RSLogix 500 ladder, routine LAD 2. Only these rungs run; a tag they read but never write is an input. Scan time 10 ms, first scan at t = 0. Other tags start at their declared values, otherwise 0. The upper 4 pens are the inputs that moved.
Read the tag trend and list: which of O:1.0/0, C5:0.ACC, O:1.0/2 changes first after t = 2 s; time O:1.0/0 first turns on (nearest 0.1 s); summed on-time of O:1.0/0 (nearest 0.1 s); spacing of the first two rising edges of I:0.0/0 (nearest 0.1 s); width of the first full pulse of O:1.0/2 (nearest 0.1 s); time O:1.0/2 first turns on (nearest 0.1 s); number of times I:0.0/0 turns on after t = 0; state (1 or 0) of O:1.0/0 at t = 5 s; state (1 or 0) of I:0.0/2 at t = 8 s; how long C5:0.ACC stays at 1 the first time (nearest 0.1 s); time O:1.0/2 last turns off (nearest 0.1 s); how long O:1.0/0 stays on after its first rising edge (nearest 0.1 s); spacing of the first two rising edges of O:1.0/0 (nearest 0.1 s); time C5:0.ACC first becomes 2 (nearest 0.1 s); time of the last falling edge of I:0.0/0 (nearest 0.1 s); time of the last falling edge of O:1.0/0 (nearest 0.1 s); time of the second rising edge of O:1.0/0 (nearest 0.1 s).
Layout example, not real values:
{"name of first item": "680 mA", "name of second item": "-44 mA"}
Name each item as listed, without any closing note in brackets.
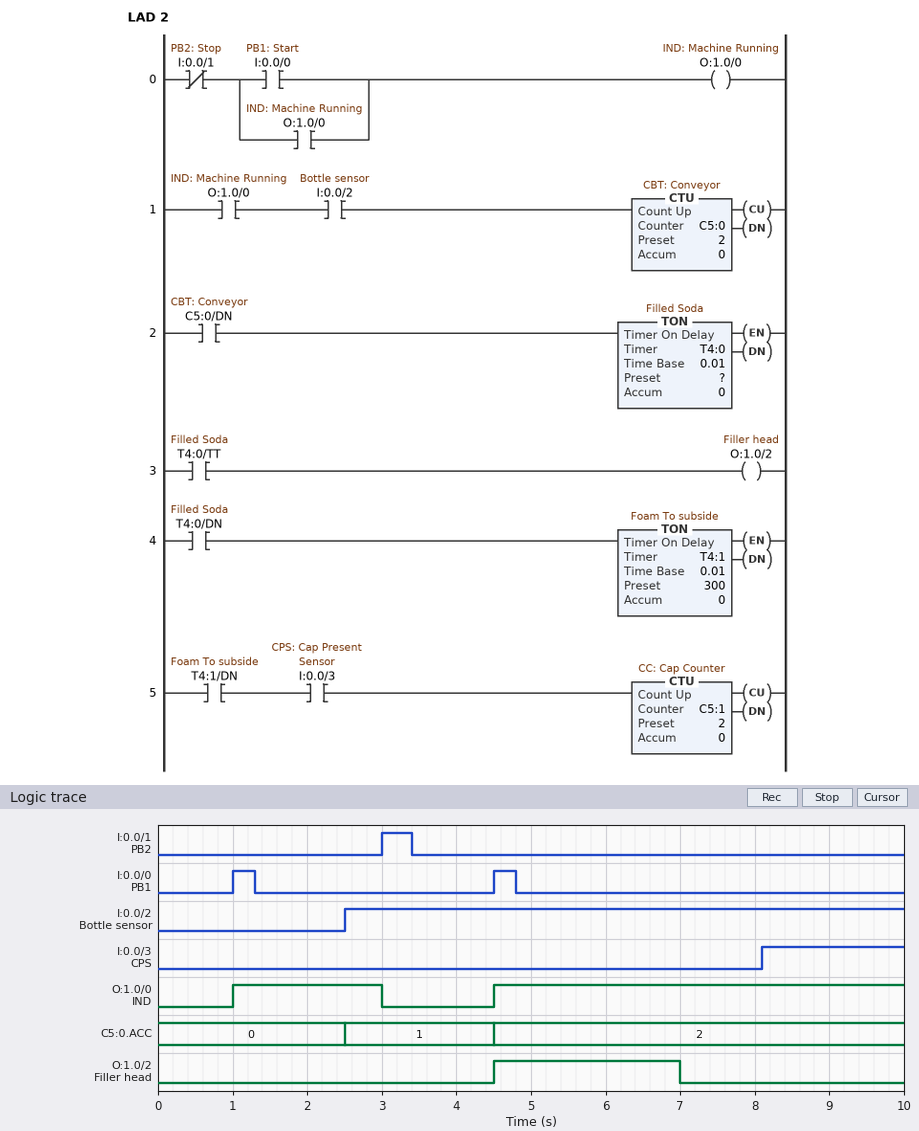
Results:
{"which of O:1.0/0, C5:0.ACC, O:1.0/2 changes first after t = 2 s": "C5:0.ACC", "time O:1.0/0 first turns on": "1.0 s", "summed on-time of O:1.0/0": "7.5 s", "spacing of the first two rising edges of I:0.0/0": "3.5 s", "width of the first full pulse of O:1.0/2": "2.5 s", "time O:1.0/2 first turns on": "4.5 s", "number of times I:0.0/0 turns on after t = 0": "2", "state (1 or 0) of O:1.0/0 at t = 5 s": "1", "state (1 or 0) of I:0.0/2 at t = 8 s": "1", "how long C5:0.ACC stays at 1 the first time": "2.0 s", "time O:1.0/2 last turns off": "7.0 s", "how long O:1.0/0 stays on after its first rising edge": "2.0 s", "spacing of the first two rising edges of O:1.0/0": "3.5 s", "time C5:0.ACC first becomes 2": "4.5 s", "time of the last falling edge of I:0.0/0": "4.8 s", "time of the last falling edge of O:1.0/0": "3.0 s", "time of the second rising edge of O:1.0/0": "4.5 s"}
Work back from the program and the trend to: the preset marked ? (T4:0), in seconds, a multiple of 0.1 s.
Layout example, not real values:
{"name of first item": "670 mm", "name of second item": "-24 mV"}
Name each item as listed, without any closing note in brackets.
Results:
{"the preset marked ? (T4:0), in seconds, a multiple of 0.1 s": "2.5 s"}
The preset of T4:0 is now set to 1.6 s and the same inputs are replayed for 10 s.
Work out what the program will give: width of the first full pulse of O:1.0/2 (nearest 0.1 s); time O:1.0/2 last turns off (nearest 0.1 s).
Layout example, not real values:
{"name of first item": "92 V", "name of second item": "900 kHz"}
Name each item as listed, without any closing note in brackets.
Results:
{"width of the first full pulse of O:1.0/2": "1.6 s", "time O:1.0/2 last turns off": "6.1 s"}
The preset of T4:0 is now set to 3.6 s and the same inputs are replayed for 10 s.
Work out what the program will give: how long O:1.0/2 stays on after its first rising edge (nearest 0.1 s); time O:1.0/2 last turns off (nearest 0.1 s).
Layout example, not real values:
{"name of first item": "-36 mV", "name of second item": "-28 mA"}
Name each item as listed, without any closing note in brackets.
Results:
{"how long O:1.0/2 stays on after its first rising edge": "3.6 s", "time O:1.0/2 last turns off": "8.1 s"}
